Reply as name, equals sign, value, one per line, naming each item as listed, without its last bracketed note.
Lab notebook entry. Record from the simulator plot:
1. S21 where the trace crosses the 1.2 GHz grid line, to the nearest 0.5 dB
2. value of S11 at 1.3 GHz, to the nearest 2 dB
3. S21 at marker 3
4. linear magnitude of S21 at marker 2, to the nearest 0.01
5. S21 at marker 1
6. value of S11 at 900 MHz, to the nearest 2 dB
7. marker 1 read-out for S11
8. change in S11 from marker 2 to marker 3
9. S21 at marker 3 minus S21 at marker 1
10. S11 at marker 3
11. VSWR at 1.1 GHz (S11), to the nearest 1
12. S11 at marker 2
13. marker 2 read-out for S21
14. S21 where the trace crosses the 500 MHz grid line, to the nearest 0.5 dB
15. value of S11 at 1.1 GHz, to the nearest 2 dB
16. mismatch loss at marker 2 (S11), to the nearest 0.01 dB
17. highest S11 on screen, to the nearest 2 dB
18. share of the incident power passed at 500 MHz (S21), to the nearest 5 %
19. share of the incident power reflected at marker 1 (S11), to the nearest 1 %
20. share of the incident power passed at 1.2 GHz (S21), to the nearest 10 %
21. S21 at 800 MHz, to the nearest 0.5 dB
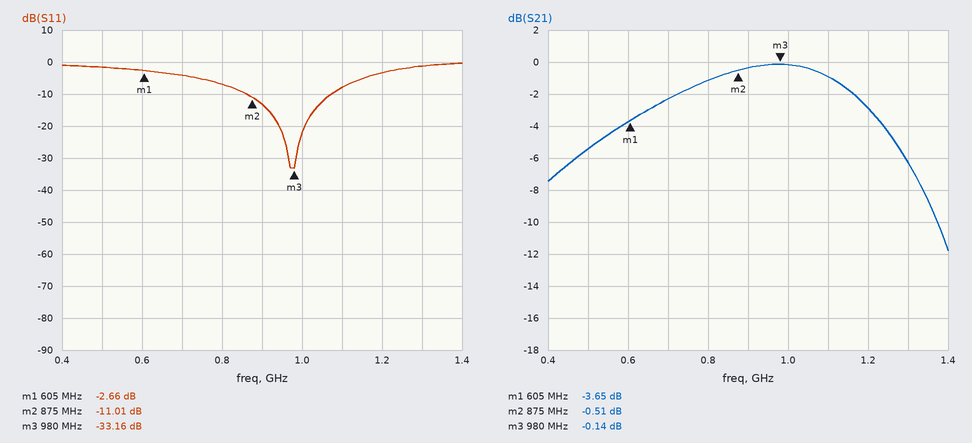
S21 where the trace crosses the 1.2 GHz grid line, to the nearest 0.5 dB = -3.0 dB
value of S11 at 1.3 GHz, to the nearest 2 dB = -2 dB
S21 at marker 3 = -0.14 dB
linear magnitude of S21 at marker 2, to the nearest 0.01 = 0.94
S21 at marker 1 = -3.65 dB
value of S11 at 900 MHz, to the nearest 2 dB = -14 dB
marker 1 read-out for S11 = -2.66 dB
change in S11 from marker 2 to marker 3 = -22.15 dB
S21 at marker 3 minus S21 at marker 1 = 3.51 dB
S11 at marker 3 = -33.16 dB
VSWR at 1.1 GHz (S11), to the nearest 1 = 2
S11 at marker 2 = -11.01 dB
marker 2 read-out for S21 = -0.51 dB
S21 where the trace crosses the 500 MHz grid line, to the nearest 0.5 dB = -5.5 dB
value of S11 at 1.1 GHz, to the nearest 2 dB = -8 dB
mismatch loss at marker 2 (S11), to the nearest 0.01 dB = 0.36 dB
highest S11 on screen, to the nearest 2 dB = 0 dB
share of the incident power passed at 500 MHz (S21), to the nearest 5 % = 30 %
share of the incident power reflected at marker 1 (S11), to the nearest 1 % = 54 %
share of the incident power passed at 1.2 GHz (S21), to the nearest 10 % = 50 %
S21 at 800 MHz, to the nearest 0.5 dB = -1.0 dB
